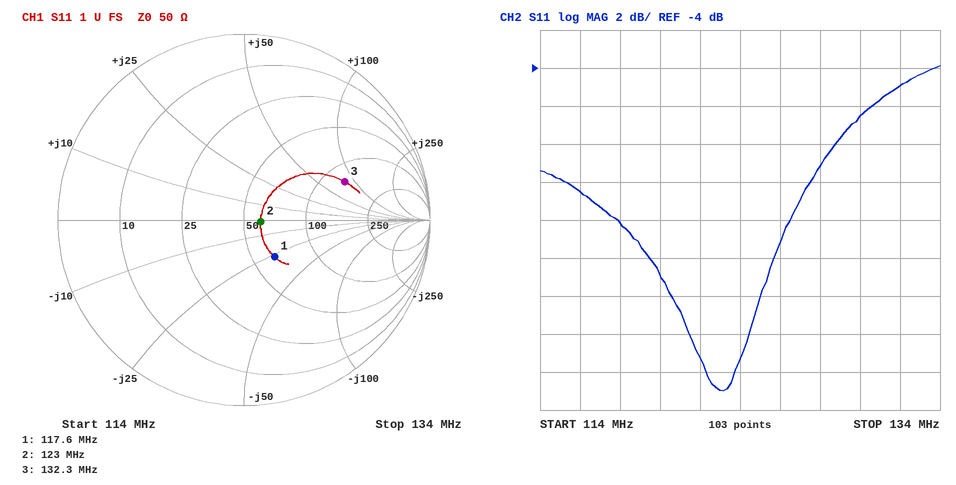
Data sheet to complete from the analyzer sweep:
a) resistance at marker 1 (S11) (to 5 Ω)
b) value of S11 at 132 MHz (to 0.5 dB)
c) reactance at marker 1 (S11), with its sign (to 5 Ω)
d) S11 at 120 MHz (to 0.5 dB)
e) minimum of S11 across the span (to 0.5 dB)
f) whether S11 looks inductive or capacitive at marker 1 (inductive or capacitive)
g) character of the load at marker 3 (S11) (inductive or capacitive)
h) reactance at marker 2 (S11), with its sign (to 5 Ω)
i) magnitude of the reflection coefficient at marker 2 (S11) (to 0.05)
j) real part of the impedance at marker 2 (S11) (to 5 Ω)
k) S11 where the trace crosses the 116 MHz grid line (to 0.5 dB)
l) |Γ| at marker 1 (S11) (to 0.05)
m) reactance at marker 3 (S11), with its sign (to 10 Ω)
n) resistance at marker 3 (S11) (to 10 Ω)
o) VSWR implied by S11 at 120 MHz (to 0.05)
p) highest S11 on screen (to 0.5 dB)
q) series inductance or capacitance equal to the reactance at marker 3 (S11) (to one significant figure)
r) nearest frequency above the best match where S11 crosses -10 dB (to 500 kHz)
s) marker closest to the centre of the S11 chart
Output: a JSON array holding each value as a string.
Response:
["65 Ω", "-5.0 dB", "-25 Ω", "-15.0 dB", "-21.0 dB", "capacitive", "inductive", "0 Ω", "0.10", "60 Ω", "-10.5 dB", "0.25", "+80 Ω", "130 Ω", "1.45", "-4.0 dB", "100 nH", "127.5 MHz", "marker 2"]
